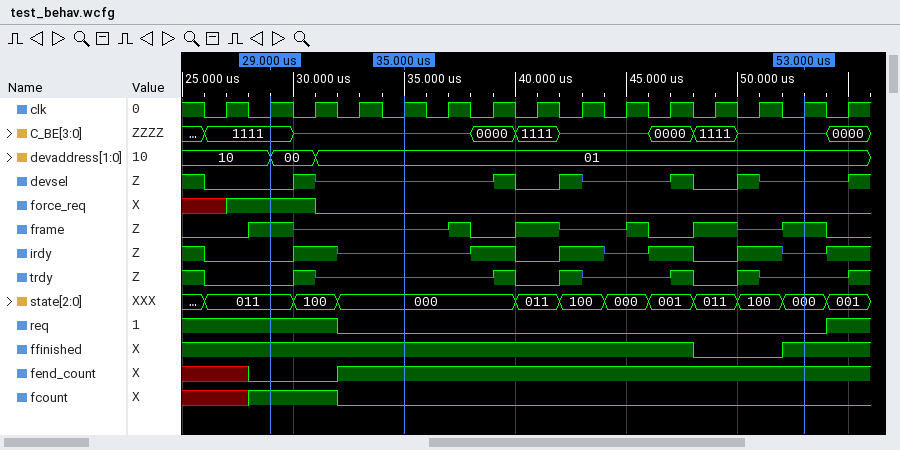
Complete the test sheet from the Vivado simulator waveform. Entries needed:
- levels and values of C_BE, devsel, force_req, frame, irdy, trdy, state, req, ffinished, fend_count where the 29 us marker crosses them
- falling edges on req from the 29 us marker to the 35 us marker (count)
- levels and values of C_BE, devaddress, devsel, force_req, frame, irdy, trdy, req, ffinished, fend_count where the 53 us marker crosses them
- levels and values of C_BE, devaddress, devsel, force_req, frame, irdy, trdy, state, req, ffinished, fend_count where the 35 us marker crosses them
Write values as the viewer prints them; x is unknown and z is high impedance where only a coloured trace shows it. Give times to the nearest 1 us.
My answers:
C_BE=1111, devsel=0, force_req=1, frame=1, irdy=0, trdy=0, state=011, req=1, ffinished=1, fend_count=0
1
C_BE=z, devaddress=01, devsel=z, force_req=0, frame=1, irdy=z, trdy=z, req=0, ffinished=1, fend_count=1
C_BE=z, devaddress=01, devsel=z, force_req=0, frame=z, irdy=z, trdy=z, state=000, req=0, ffinished=1, fend_count=1
